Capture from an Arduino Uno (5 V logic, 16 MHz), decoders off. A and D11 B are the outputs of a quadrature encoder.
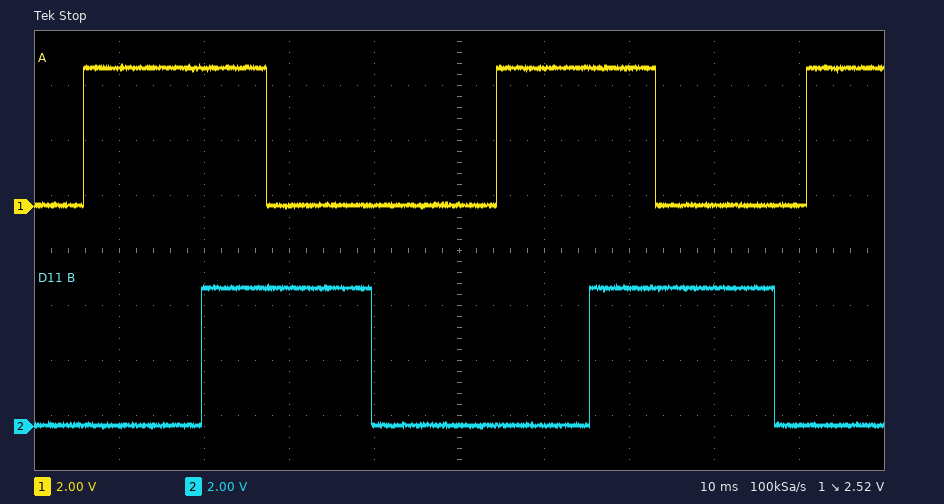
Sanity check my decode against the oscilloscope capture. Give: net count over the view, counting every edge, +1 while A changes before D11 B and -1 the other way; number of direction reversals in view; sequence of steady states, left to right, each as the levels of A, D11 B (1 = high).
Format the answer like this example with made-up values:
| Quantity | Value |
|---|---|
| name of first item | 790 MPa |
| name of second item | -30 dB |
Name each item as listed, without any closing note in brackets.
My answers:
| Quantity | Value |
|---|---|
| net count over the view, counting every edge, +1 while A changes before D11 B and -1 the other way | +9 |
| number of direction reversals in view | 0 |
| sequence of steady states, left to right, each as the levels of A, D11 B | 00 10 11 01 00 10 11 01 00 10 |
